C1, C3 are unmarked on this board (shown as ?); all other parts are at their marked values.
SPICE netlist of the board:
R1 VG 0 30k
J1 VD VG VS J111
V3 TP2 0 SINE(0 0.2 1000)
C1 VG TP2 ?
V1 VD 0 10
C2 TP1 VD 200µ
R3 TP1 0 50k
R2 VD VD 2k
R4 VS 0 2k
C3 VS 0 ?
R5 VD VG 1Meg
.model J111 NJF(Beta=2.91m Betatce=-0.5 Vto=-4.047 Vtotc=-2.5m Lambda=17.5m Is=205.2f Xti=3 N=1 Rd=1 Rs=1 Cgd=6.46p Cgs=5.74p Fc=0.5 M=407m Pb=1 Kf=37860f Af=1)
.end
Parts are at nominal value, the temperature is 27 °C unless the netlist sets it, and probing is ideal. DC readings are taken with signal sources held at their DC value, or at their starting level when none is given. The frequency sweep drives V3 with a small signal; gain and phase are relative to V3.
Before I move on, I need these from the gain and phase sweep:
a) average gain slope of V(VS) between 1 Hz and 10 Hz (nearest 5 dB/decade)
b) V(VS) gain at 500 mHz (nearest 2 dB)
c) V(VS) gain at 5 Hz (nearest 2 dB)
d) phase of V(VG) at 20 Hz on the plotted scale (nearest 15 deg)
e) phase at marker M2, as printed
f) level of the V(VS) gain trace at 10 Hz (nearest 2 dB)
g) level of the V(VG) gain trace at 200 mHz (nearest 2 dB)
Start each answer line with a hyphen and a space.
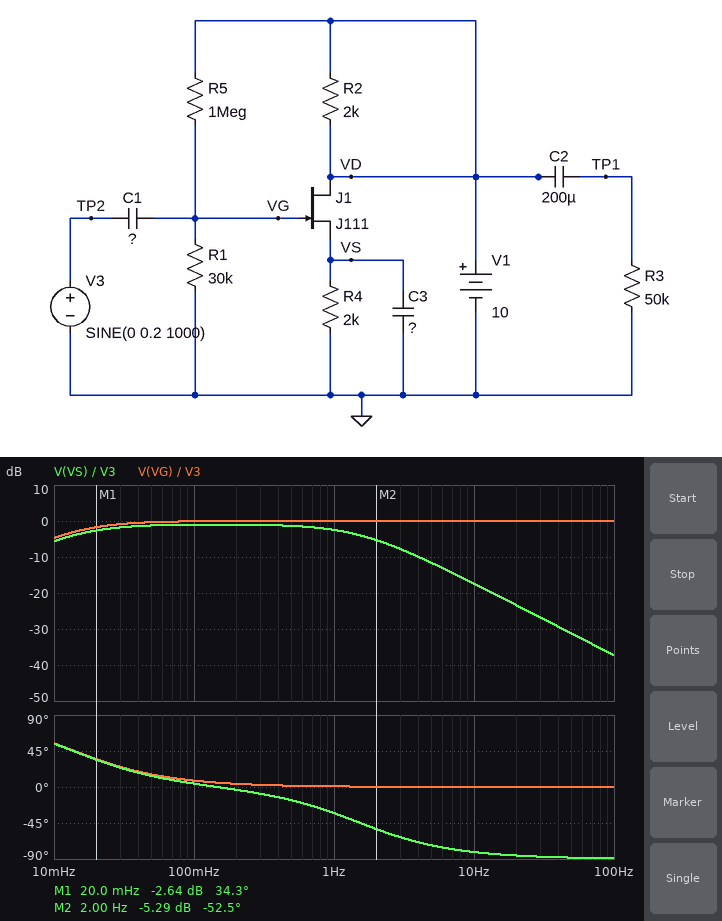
- -15 dB/decade
- -2 dB
- -12 dB
- 0 deg
- -52.5 deg
- -18 dB
- 0 dB
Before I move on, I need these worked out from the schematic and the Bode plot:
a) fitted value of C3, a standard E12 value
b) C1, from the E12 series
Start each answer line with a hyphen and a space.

- 560 µF
- 390 µF
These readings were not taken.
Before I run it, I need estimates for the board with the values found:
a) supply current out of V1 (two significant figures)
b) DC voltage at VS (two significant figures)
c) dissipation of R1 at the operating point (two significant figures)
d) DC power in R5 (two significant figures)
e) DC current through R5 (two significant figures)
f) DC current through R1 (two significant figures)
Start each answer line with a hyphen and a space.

- 1.8 mA
- 3.6 V
- 2.8 µW
- 94 µW
- 9.7 µA
- 9.7 µA
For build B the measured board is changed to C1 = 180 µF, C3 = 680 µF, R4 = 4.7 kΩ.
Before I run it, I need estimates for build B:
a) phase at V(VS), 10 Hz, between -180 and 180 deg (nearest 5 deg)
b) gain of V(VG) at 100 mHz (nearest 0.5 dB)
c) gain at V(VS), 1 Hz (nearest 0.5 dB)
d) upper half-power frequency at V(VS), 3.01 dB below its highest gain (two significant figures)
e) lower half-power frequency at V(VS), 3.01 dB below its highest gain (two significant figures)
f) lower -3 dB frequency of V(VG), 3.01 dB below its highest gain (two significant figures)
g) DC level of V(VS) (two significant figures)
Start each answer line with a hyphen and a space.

- -85 deg
- -0.5 dB
- -4.5 dB
- 870 mHz
- 28 mHz
- 30 mHz
- 3.8 V
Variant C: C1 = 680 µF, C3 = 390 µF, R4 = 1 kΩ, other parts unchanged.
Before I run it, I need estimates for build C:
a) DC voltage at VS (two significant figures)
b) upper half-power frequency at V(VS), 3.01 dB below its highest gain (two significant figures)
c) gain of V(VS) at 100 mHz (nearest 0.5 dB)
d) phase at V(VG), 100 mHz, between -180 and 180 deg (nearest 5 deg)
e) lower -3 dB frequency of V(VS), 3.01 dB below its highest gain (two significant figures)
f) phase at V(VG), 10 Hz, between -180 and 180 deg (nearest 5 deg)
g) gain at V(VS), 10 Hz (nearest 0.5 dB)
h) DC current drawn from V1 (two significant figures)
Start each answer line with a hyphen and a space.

- 3.3 V
- 3.1 Hz
- -1.5 dB
- 5 deg
- 8.0 mHz
- 0 deg
- -12.0 dB
- 3.3 mA
